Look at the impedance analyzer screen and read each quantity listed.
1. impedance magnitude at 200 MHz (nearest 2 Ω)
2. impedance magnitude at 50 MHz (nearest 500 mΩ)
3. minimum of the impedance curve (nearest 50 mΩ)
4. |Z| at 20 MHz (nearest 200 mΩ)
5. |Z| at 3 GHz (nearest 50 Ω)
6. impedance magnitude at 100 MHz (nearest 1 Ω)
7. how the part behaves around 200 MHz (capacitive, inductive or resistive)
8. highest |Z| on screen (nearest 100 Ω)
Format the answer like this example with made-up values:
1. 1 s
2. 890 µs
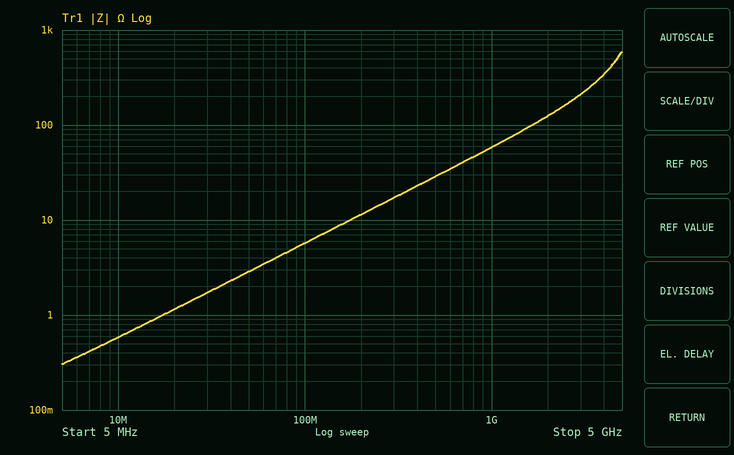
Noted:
1. 12 Ω
2. 3.0 Ω
3. 300 mΩ
4. 1.2 Ω
5. 200 Ω
6. 6 Ω
7. inductive
8. 600 Ω
